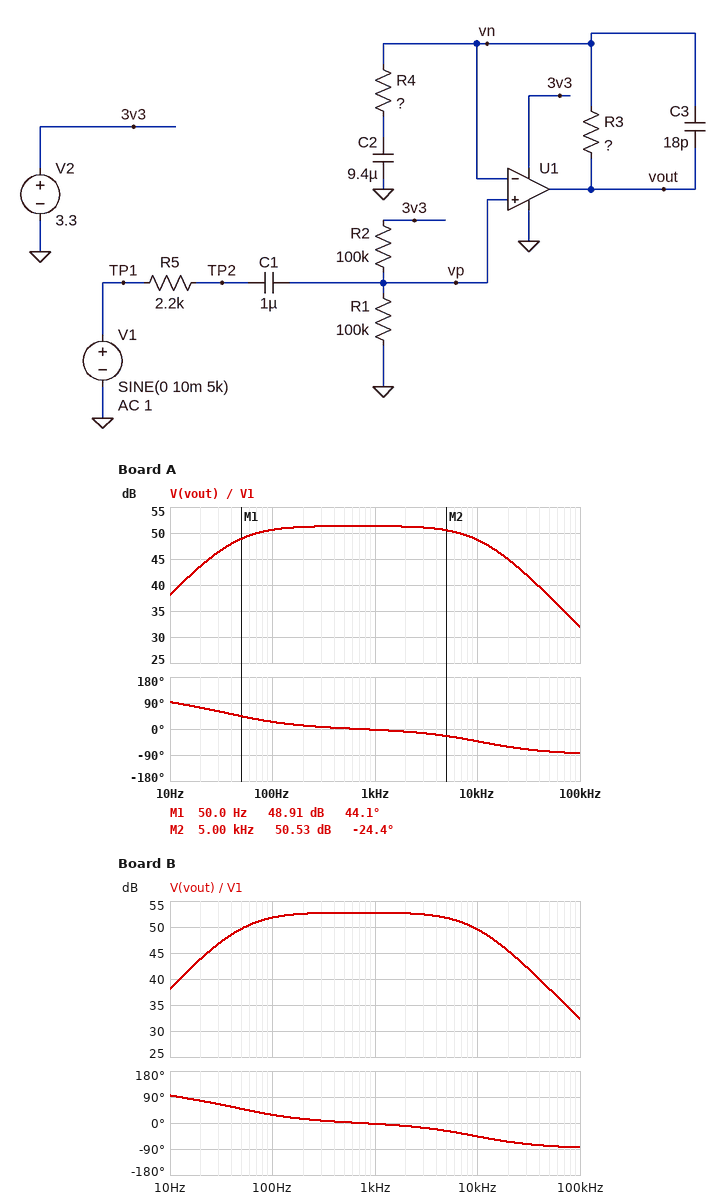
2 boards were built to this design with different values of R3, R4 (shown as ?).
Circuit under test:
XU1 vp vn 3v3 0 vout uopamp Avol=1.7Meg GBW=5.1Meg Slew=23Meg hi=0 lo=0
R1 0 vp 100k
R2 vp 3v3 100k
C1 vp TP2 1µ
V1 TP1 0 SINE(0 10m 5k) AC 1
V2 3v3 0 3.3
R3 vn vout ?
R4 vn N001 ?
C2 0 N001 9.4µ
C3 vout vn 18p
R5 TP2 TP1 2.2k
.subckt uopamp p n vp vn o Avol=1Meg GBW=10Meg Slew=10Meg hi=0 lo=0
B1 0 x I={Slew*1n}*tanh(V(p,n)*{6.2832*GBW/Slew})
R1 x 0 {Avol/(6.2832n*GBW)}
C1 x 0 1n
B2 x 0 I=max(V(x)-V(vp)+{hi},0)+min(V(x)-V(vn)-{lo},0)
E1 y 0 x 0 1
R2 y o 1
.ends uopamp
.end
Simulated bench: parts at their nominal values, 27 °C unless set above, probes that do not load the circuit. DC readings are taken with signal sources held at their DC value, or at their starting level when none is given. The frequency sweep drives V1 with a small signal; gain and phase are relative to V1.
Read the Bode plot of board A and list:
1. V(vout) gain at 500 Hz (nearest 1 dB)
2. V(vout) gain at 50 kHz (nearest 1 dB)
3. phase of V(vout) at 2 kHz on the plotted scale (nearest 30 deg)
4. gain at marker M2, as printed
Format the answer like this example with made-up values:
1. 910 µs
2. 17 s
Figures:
1. 51 dB
2. 38 dB
3. 0 deg
4. 50.53 dB
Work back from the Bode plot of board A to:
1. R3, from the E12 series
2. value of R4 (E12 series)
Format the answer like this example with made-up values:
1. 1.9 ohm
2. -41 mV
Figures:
1. 150 kΩ
2. 390 Ω
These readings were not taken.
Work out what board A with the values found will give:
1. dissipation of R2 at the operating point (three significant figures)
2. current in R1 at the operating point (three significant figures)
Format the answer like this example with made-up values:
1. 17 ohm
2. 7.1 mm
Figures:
1. 27.2 µW
2. 16.5 µA
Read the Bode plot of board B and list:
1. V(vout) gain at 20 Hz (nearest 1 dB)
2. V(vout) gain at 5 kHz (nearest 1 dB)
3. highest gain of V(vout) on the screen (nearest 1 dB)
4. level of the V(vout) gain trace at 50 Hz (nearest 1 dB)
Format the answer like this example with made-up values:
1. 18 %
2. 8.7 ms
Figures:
1. 44 dB
2. 52 dB
3. 53 dB
4. 50 dB
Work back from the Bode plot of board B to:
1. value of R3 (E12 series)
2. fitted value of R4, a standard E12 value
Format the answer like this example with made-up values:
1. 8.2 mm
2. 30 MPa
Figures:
1. 150 kΩ
2. 330 Ω
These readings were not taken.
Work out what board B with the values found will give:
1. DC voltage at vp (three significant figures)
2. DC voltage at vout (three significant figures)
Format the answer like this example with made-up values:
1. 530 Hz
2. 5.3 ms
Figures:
1. 1.65 V
2. 1.65 V
